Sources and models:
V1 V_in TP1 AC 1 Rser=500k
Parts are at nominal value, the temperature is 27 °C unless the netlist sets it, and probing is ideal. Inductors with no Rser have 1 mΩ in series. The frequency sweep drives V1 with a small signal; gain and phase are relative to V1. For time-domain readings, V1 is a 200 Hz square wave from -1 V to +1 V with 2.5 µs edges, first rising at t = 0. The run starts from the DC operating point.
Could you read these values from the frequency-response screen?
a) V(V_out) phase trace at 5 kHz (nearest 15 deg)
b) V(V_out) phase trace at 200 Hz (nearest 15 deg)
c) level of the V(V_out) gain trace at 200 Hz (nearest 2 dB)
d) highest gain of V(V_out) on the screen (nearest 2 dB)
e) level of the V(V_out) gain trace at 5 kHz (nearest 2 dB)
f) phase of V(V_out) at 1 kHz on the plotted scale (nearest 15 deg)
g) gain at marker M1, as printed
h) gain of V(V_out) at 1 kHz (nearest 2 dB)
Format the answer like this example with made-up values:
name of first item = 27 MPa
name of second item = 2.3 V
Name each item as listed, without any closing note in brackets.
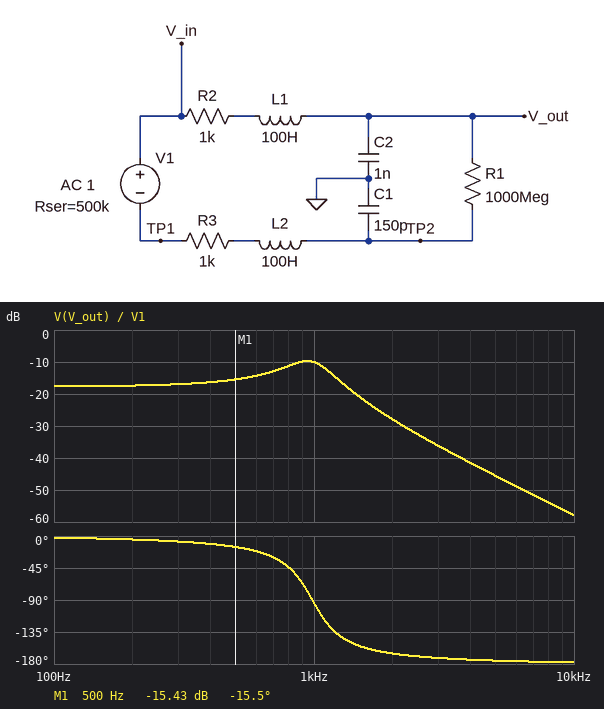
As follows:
V(V_out) phase trace at 5 kHz = -180 deg
V(V_out) phase trace at 200 Hz = 0 deg
level of the V(V_out) gain trace at 200 Hz = -18 dB
highest gain of V(V_out) on the screen = -10 dB
level of the V(V_out) gain trace at 5 kHz = -46 dB
phase of V(V_out) at 1 kHz on the plotted scale = -90 deg
gain at marker M1, as printed = -15.43 dB
gain of V(V_out) at 1 kHz = -10 dB
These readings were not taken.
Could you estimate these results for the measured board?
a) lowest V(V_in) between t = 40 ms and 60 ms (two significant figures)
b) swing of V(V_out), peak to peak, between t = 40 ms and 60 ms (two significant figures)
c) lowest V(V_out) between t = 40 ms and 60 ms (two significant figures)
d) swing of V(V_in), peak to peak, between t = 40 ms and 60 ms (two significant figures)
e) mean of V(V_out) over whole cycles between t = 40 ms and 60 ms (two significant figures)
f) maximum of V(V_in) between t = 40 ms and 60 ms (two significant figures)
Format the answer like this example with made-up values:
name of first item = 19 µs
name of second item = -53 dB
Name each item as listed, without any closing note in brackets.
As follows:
lowest V(V_in) between t = 40 ms and 60 ms = -1.3 V
swing of V(V_out), peak to peak, between t = 40 ms and 60 ms = 540 mV
lowest V(V_out) between t = 40 ms and 60 ms = -640 mV
swing of V(V_in), peak to peak, between t = 40 ms and 60 ms = 1.8 V
mean of V(V_out) over whole cycles between t = 40 ms and 60 ms = -370 mV
maximum of V(V_in) between t = 40 ms and 60 ms = 530 mV
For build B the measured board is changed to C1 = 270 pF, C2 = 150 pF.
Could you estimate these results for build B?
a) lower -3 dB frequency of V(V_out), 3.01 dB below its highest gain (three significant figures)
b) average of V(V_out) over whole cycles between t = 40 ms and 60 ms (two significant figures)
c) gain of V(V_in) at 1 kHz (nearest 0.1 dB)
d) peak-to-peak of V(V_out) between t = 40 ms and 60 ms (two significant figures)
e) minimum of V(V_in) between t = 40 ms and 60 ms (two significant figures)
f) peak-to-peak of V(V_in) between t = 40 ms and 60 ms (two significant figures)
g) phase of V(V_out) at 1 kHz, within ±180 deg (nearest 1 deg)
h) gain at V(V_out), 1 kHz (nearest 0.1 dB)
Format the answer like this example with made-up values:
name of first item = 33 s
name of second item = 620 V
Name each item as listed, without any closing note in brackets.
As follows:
lower -3 dB frequency of V(V_out), 3.01 dB below its highest gain = 884 Hz
average of V(V_out) over whole cycles between t = 40 ms and 60 ms = 140 mV
gain of V(V_in) at 1 kHz = -3.4 dB
peak-to-peak of V(V_out) between t = 40 ms and 60 ms = 2.7 V
minimum of V(V_in) between t = 40 ms and 60 ms = -740 mV
peak-to-peak of V(V_in) between t = 40 ms and 60 ms = 1.8 V
phase of V(V_out) at 1 kHz, within ±180 deg = -52 deg
gain at V(V_out), 1 kHz = 4.4 dB
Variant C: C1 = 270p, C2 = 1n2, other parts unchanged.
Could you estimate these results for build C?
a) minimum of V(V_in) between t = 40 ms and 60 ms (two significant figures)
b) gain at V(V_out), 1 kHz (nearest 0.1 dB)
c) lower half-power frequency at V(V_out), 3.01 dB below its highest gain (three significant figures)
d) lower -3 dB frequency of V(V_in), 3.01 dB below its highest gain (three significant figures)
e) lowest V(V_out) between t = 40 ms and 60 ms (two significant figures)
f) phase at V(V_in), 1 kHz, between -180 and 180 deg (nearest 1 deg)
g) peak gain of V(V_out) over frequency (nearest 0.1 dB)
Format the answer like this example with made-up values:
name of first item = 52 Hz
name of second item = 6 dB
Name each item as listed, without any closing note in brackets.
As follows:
minimum of V(V_in) between t = 40 ms and 60 ms = -1.1 V
gain at V(V_out), 1 kHz = -14.9 dB
lower half-power frequency at V(V_out), 3.01 dB below its highest gain = 450 Hz
lower -3 dB frequency of V(V_in), 3.01 dB below its highest gain = 707 Hz
lowest V(V_out) between t = 40 ms and 60 ms = -650 mV
phase at V(V_in), 1 kHz, between -180 and 180 deg = 43 deg
peak gain of V(V_out) over frequency = -8.9 dB
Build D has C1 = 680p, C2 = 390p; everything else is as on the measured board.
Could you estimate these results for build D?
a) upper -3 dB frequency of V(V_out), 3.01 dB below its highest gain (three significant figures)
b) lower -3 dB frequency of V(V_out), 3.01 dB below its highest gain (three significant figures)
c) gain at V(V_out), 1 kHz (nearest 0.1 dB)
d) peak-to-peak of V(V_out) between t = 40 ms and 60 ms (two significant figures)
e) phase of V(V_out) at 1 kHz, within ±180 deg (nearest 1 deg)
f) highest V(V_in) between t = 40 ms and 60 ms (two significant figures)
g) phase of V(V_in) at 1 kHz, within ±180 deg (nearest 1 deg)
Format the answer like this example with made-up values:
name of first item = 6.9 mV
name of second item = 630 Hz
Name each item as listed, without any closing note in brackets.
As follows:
upper -3 dB frequency of V(V_out), 3.01 dB below its highest gain = 840 Hz
lower -3 dB frequency of V(V_out), 3.01 dB below its highest gain = 396 Hz
gain at V(V_out), 1 kHz = -5.8 dB
peak-to-peak of V(V_out) between t = 40 ms and 60 ms = 2.3 V
phase of V(V_out) at 1 kHz, within ±180 deg = -141 deg
highest V(V_in) between t = 40 ms and 60 ms = 990 mV
phase of V(V_in) at 1 kHz, within ±180 deg = 39 deg
